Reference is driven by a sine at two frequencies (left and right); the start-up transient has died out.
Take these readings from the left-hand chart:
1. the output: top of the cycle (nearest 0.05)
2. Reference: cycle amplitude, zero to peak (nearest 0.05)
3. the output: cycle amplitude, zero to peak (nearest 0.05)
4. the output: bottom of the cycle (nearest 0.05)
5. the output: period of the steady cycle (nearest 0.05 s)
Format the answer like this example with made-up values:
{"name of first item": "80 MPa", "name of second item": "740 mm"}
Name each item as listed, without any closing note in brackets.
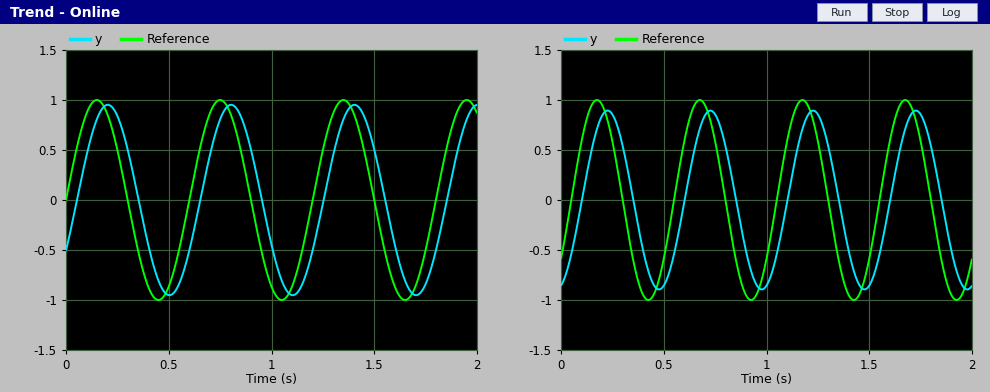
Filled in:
{"the output: top of the cycle": "0.95", "Reference: cycle amplitude, zero to peak": "1.00", "the output: cycle amplitude, zero to peak": "0.95", "the output: bottom of the cycle": "-0.95", "the output: period of the steady cycle": "0.60 s"}
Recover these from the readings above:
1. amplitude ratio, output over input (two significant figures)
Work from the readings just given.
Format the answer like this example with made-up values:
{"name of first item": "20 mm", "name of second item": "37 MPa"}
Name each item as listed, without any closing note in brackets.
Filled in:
{"amplitude ratio, output over input": "0.95"}
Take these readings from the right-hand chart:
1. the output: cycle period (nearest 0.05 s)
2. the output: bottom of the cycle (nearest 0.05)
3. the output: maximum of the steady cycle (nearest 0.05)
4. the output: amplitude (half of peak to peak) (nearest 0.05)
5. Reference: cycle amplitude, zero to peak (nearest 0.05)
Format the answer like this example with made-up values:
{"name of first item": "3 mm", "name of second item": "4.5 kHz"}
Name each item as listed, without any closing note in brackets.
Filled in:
{"the output: cycle period": "0.50 s", "the output: bottom of the cycle": "-0.90", "the output: maximum of the steady cycle": "0.90", "the output: amplitude (half of peak to peak)": "0.90", "Reference: cycle amplitude, zero to peak": "1.00"}
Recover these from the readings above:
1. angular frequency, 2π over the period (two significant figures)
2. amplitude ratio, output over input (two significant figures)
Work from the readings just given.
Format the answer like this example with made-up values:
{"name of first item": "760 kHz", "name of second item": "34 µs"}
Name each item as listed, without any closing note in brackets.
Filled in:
{"angular frequency, 2π over the period": "13 rad/s", "amplitude ratio, output over input": "0.90"}
